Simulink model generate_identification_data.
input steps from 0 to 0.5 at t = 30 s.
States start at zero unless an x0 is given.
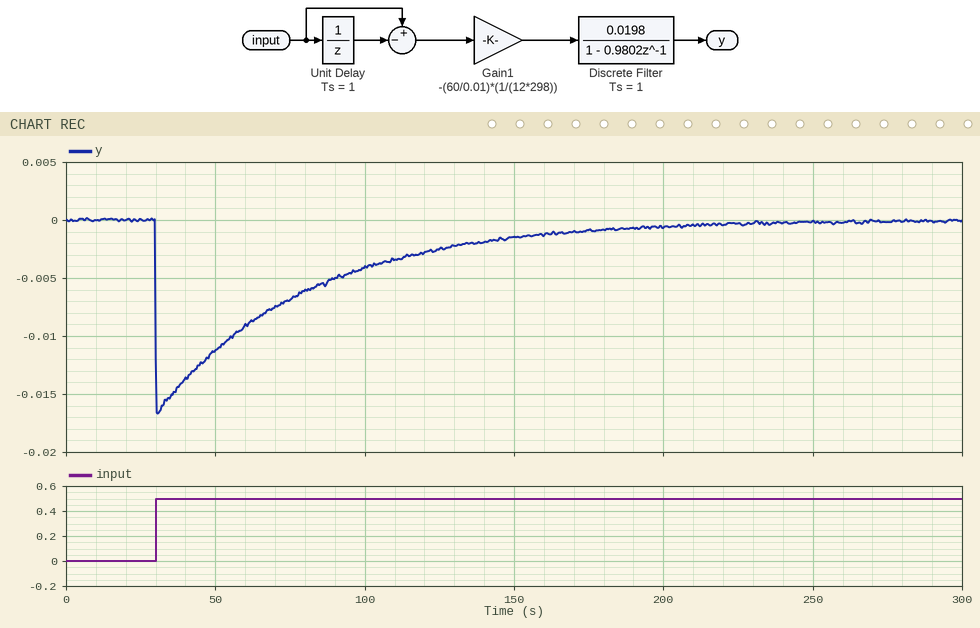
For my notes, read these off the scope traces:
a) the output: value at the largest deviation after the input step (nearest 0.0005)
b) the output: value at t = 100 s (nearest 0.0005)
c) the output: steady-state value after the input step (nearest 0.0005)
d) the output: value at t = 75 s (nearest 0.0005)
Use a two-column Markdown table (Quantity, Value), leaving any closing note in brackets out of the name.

| Quantity | Value |
|---|---|
| the output: value at the largest deviation after the input step | -0.0165 |
| the output: value at t = 100 s | -0.0040 |
| the output: steady-state value after the input step | 0.0000 |
| the output: value at t = 75 s | -0.0070 |
